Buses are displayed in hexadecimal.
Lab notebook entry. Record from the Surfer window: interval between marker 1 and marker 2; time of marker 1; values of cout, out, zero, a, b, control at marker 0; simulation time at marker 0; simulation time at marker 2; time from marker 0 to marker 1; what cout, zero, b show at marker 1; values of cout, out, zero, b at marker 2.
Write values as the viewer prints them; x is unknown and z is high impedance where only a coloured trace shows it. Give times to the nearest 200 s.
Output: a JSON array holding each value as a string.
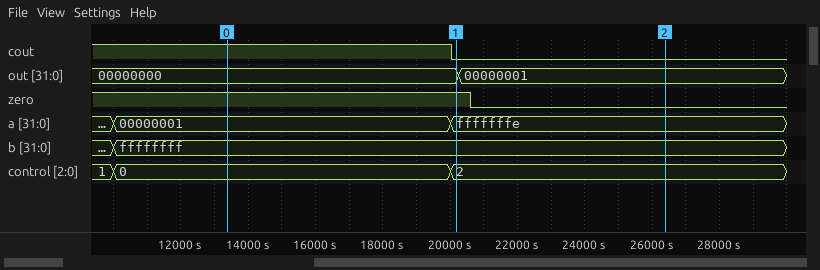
["6200 s", "20200 s", "cout=1, out=00000000, zero=1, a=00000001, b=ffffffff, control=0", "13400 s", "26400 s", "6800 s", "cout=0, zero=1, b=ffffffff", "cout=0, out=00000001, zero=0, b=ffffffff"]
